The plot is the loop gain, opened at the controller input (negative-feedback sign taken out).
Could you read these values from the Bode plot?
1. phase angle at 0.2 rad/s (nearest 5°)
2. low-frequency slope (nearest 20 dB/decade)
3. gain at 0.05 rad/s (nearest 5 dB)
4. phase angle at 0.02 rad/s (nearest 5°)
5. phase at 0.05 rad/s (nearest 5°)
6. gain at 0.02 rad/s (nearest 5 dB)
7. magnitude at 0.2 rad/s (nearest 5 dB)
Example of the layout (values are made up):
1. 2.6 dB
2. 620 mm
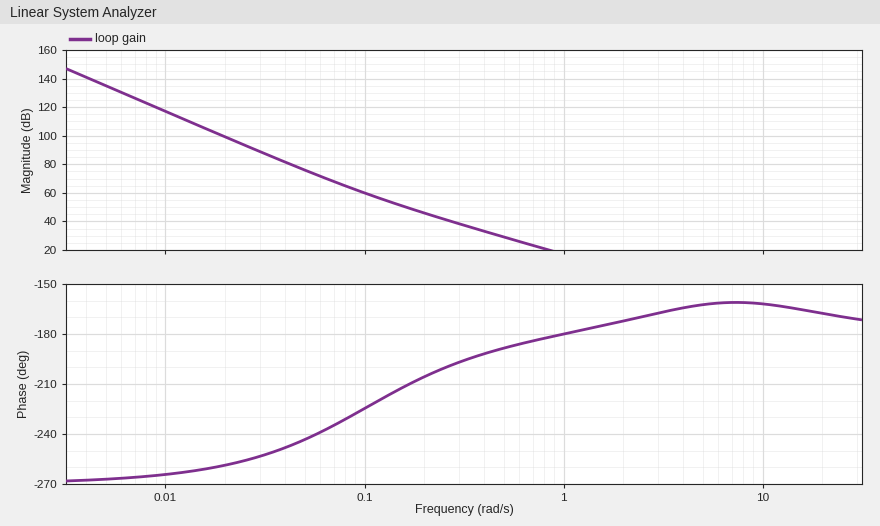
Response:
1. -205°
2. -60 dB/decade
3. 75 dB
4. -260°
5. -245°
6. 100 dB
7. 45 dB
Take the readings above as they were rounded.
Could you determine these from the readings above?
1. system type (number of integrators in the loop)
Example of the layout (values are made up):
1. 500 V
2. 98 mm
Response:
1. 3
